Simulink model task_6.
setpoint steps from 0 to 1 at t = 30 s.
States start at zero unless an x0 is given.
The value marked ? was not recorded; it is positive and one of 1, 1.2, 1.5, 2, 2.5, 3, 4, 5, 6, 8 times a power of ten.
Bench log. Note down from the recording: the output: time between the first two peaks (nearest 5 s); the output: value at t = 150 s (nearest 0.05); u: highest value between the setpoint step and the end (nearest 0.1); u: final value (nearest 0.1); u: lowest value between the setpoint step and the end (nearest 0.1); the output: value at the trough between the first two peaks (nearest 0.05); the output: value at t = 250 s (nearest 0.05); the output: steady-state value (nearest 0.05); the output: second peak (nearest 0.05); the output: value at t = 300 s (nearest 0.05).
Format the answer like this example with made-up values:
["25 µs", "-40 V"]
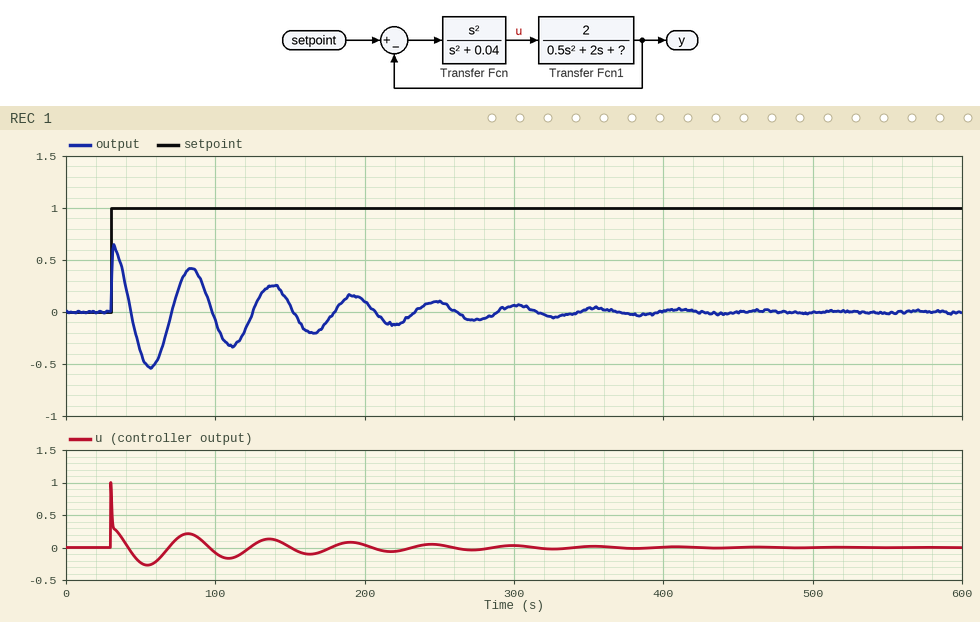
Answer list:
["50 s", "0.05", "1.0", "0.0", "-0.3", "-0.55", "0.10", "0.00", "0.40", "0.05"]
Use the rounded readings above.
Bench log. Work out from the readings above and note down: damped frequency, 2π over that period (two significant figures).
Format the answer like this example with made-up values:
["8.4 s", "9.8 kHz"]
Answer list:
["0.13 rad/s"]
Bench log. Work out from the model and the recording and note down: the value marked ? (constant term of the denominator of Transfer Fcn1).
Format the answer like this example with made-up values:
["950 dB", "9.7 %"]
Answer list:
["1"]
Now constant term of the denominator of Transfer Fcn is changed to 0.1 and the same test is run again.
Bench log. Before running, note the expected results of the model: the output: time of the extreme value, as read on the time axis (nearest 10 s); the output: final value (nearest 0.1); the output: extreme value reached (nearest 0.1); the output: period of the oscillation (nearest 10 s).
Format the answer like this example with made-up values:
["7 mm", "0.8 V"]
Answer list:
["30 s", "0.0", "0.6", "30 s"]
